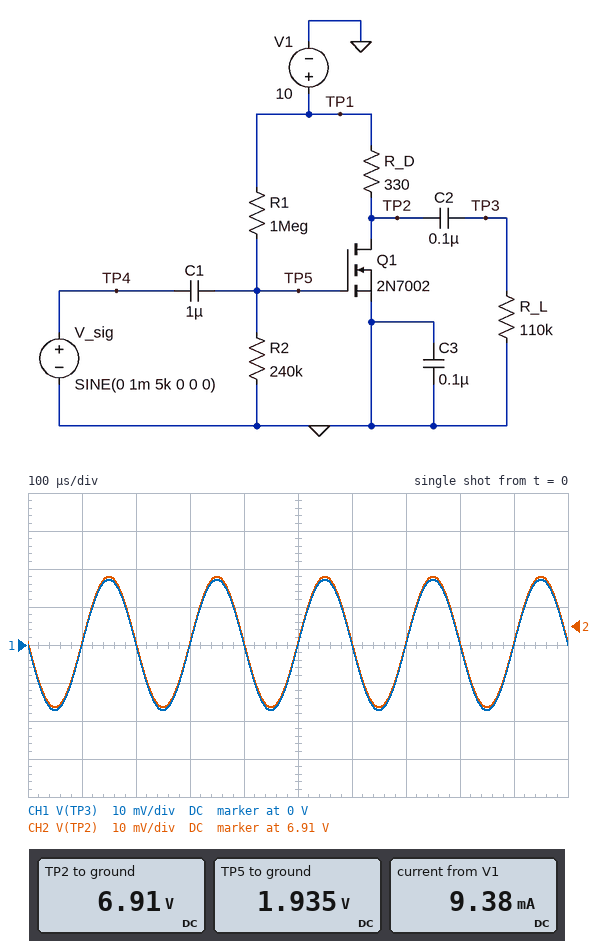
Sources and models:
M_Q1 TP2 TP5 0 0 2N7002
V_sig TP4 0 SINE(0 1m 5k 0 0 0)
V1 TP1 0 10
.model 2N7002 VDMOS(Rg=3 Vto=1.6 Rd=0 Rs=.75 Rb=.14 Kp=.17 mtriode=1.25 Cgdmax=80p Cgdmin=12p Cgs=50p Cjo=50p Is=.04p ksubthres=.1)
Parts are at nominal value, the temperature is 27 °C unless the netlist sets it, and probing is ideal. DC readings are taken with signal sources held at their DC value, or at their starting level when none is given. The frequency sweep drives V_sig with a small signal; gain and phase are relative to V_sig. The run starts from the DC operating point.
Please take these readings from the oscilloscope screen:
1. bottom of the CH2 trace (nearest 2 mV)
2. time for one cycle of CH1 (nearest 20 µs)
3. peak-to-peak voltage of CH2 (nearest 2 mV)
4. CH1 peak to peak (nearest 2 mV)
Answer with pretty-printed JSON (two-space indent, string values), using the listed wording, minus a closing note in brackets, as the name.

{
  "bottom of the CH2 trace": "6.888 V",
  "time for one cycle of CH1": "200 µs",
  "peak-to-peak voltage of CH2": "34 mV",
  "CH1 peak to peak": "34 mV"
}
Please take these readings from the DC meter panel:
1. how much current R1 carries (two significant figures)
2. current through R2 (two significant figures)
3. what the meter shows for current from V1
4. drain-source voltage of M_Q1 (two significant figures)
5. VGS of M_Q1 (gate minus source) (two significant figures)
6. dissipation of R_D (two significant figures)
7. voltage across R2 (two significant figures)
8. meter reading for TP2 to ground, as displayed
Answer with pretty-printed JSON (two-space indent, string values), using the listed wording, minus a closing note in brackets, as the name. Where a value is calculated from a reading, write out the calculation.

{
  "how much current R1 carries": "(10 V - 1.935 V) / 1 MΩ = 8.1 µA",
  "current through R2": "(1.935 V) / 240 kΩ = 8.1 µA",
  "what the meter shows for current from V1": "9.38 mA",
  "drain-source voltage of M_Q1": "6.91 V = 6.9 V",
  "VGS of M_Q1 (gate minus source)": "1.935 V = 1.9 V",
  "dissipation of R_D": "(10 V - 6.91 V)^2 / 330 Ω = 29 mW",
  "voltage across R2": "1.935 V = 1.9 V",
  "meter reading for TP2 to ground, as displayed": "6.91 V"
}
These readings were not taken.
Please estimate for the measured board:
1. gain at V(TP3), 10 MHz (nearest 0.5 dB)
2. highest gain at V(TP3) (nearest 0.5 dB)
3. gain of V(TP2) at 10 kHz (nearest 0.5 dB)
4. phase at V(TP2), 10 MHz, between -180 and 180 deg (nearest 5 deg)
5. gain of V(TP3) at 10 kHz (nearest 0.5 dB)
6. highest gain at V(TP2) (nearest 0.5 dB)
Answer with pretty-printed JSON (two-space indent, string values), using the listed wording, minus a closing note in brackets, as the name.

{
  "gain at V(TP3), 10 MHz": "23.0 dB",
  "highest gain at V(TP3)": "24.5 dB",
  "gain of V(TP2) at 10 kHz": "24.5 dB",
  "phase at V(TP2), 10 MHz, between -180 and 180 deg": "140 deg",
  "gain of V(TP3) at 10 kHz": "24.5 dB",
  "highest gain at V(TP2)": "24.5 dB"
}
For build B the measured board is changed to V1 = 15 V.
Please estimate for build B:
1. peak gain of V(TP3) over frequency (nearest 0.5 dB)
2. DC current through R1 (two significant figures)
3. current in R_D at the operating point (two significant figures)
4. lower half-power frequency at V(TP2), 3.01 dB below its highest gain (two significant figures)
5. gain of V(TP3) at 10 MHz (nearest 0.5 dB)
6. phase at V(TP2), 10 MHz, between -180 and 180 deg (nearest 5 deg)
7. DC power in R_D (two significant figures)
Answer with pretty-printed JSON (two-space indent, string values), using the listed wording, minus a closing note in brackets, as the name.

{
  "peak gain of V(TP3) over frequency": "-7.5 dB",
  "DC current through R1": "12 µA",
  "current in R_D at the operating point": "45 mA",
  "lower half-power frequency at V(TP2), 3.01 dB below its highest gain": "110 MHz",
  "gain of V(TP3) at 10 MHz": "-15.0 dB",
  "phase at V(TP2), 10 MHz, between -180 and 180 deg": "165 deg",
  "DC power in R_D": "660 mW"
}
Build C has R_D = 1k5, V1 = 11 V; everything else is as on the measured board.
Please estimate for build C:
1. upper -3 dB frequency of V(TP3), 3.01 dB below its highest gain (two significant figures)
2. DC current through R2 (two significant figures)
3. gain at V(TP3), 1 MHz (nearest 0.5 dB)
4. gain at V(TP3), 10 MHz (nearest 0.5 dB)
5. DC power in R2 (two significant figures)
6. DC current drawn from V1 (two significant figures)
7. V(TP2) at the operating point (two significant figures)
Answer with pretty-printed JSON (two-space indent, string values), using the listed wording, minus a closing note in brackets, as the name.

{
  "upper -3 dB frequency of V(TP3), 3.01 dB below its highest gain": "910 MHz",
  "DC current through R2": "8.9 µA",
  "gain at V(TP3), 1 MHz": "-16.0 dB",
  "gain at V(TP3), 10 MHz": "-15.5 dB",
  "DC power in R2": "19 µW",
  "DC current drawn from V1": "7.3 mA",
  "V(TP2) at the operating point": "77 mV"
}
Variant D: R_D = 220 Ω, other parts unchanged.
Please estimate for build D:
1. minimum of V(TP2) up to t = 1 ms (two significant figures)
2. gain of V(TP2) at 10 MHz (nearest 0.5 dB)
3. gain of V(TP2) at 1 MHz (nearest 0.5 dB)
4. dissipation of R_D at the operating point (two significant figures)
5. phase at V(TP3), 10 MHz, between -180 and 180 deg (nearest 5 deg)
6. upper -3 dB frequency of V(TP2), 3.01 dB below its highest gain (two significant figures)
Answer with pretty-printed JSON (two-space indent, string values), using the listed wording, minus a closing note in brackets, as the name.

{
  "minimum of V(TP2) up to t = 1 ms": "7.9 V",
  "gain of V(TP2) at 10 MHz": "20.5 dB",
  "gain of V(TP2) at 1 MHz": "21.0 dB",
  "dissipation of R_D at the operating point": "19 mW",
  "phase at V(TP3), 10 MHz, between -180 and 180 deg": "155 deg",
  "upper -3 dB frequency of V(TP2), 3.01 dB below its highest gain": "21 MHz"
}
